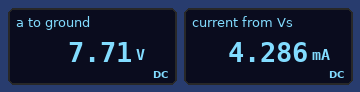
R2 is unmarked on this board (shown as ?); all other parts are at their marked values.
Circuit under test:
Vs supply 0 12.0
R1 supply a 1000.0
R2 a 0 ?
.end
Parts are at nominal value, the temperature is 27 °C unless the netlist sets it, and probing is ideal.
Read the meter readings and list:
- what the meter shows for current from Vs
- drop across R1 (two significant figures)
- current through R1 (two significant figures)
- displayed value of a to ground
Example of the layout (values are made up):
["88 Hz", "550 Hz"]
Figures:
["4.286 mA", "4.3 V", "4.3 mA", "7.71 V"]
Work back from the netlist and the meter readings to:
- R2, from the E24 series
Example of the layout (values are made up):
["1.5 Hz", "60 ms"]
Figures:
["1.8 kΩ"]
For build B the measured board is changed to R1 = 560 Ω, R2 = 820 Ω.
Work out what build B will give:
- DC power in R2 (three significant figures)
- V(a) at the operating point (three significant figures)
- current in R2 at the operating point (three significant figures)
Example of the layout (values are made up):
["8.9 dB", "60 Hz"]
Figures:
["62.0 mW", "7.13 V", "8.70 mA"]
